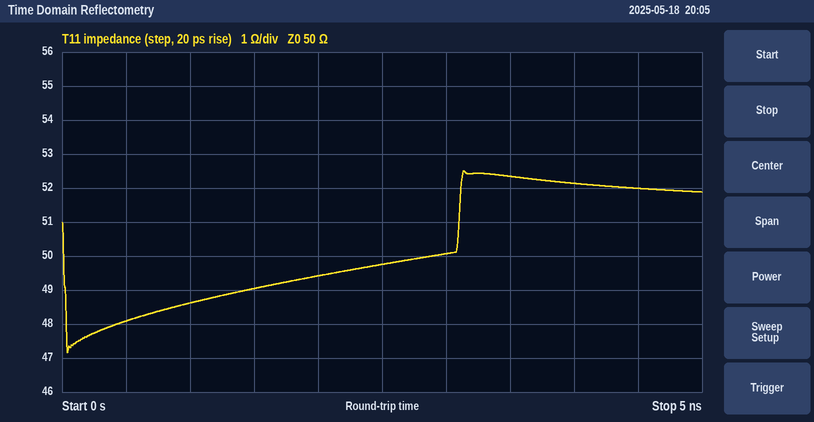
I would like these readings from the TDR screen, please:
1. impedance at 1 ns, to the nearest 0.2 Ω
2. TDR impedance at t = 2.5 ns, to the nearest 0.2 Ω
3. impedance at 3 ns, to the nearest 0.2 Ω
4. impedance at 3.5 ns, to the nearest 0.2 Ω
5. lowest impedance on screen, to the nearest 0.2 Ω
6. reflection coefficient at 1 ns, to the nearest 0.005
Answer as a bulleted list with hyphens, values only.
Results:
- 48.6 Ω
- 49.8 Ω
- 50.0 Ω
- 52.4 Ω
- 47.2 Ω
- -0.015
